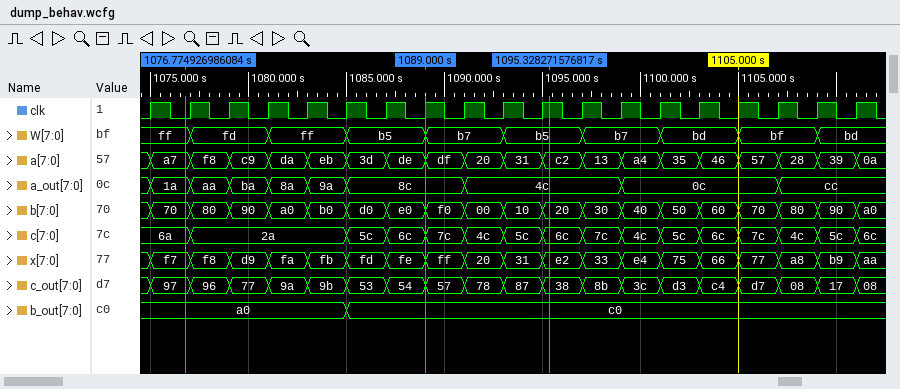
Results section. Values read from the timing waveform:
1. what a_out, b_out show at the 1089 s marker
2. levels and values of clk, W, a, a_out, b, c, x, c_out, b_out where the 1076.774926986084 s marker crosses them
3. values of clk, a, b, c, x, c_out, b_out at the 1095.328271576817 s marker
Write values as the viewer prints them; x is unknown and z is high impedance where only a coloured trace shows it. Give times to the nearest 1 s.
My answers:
a_out=8c, b_out=c0
clk=0, W=ff, a=a7, a_out=1a, b=70, c=6a, x=f7, c_out=97, b_out=a0
clk=1, a=c2, b=20, c=6c, x=e2, c_out=38, b_out=c0
